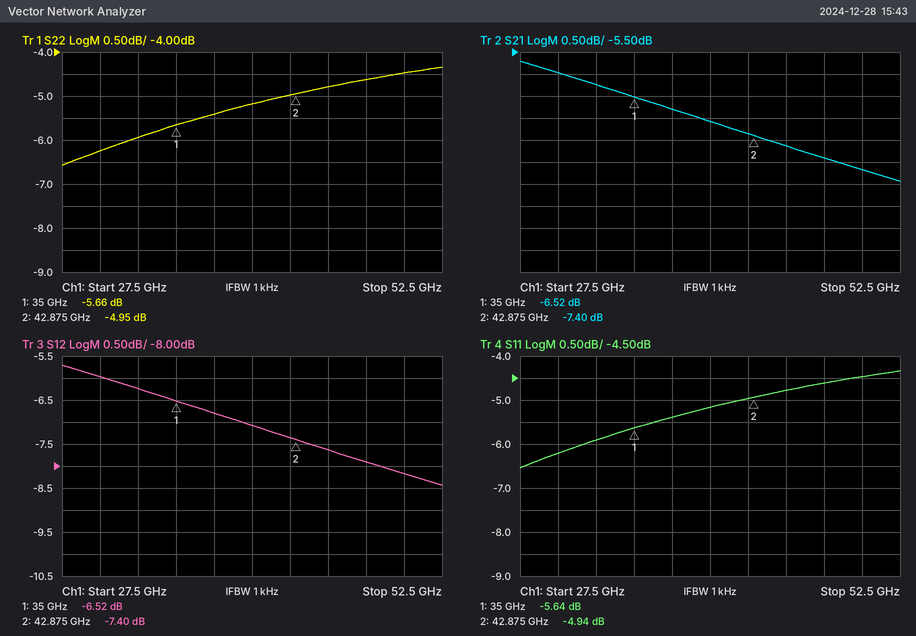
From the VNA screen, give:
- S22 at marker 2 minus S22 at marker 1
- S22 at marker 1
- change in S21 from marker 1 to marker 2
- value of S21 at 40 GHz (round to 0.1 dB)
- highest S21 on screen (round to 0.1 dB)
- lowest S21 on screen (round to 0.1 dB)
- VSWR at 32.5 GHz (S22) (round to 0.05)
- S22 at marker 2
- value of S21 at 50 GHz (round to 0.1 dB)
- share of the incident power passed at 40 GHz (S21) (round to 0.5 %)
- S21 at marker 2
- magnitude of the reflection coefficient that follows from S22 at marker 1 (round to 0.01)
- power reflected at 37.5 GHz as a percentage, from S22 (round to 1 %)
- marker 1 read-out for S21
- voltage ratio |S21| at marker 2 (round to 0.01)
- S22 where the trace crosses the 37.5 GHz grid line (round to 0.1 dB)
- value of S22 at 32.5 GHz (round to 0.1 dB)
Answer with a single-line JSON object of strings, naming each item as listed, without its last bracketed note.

{"S22 at marker 2 minus S22 at marker 1": "0.71 dB", "S22 at marker 1": "-5.66 dB", "change in S21 from marker 1 to marker 2": "-0.88 dB", "value of S21 at 40 GHz": "-7.1 dB", "highest S21 on screen": "-5.7 dB", "lowest S21 on screen": "-8.4 dB", "VSWR at 32.5 GHz (S22)": "3.05", "S22 at marker 2": "-4.95 dB", "value of S21 at 50 GHz": "-8.2 dB", "share of the incident power passed at 40 GHz (S21)": "19.5 %", "S21 at marker 2": "-7.40 dB", "magnitude of the reflection coefficient that follows from S22 at marker 1": "0.52", "power reflected at 37.5 GHz as a percentage, from S22": "29 %", "marker 1 read-out for S21": "-6.52 dB", "voltage ratio |S21| at marker 2": "0.43", "S22 where the trace crosses the 37.5 GHz grid line": "-5.4 dB", "value of S22 at 32.5 GHz": "-5.9 dB"}
